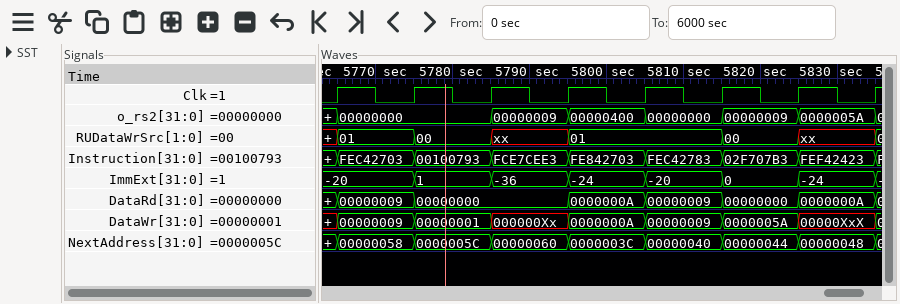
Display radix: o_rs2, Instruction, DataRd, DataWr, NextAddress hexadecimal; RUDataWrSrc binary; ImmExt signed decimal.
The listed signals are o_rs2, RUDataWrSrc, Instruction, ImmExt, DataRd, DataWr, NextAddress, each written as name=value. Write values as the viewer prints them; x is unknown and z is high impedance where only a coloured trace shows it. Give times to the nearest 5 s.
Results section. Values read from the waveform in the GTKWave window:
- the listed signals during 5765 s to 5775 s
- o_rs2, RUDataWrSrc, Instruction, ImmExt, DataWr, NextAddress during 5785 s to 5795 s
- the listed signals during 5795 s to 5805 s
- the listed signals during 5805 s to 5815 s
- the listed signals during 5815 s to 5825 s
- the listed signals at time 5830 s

o_rs2=00000000, RUDataWrSrc=01, Instruction=FEC42703, ImmExt=-20, DataRd=00000009, DataWr=00000009, NextAddress=00000058
o_rs2=00000009, RUDataWrSrc=xx, Instruction=FCE7CEE3, ImmExt=-36, DataWr=000000Xx, NextAddress=00000060
o_rs2=00000400, RUDataWrSrc=01, Instruction=FE842703, ImmExt=-24, DataRd=0000000A, DataWr=0000000A, NextAddress=0000003C
o_rs2=00000000, RUDataWrSrc=01, Instruction=FEC42783, ImmExt=-20, DataRd=00000009, DataWr=00000009, NextAddress=00000040
o_rs2=00000009, RUDataWrSrc=00, Instruction=02F707B3, ImmExt=0, DataRd=00000000, DataWr=0000005A, NextAddress=00000044
o_rs2=0000005A, RUDataWrSrc=xx, Instruction=FEF42423, ImmExt=-24, DataRd=0000000A, DataWr=00000XxX, NextAddress=00000048
